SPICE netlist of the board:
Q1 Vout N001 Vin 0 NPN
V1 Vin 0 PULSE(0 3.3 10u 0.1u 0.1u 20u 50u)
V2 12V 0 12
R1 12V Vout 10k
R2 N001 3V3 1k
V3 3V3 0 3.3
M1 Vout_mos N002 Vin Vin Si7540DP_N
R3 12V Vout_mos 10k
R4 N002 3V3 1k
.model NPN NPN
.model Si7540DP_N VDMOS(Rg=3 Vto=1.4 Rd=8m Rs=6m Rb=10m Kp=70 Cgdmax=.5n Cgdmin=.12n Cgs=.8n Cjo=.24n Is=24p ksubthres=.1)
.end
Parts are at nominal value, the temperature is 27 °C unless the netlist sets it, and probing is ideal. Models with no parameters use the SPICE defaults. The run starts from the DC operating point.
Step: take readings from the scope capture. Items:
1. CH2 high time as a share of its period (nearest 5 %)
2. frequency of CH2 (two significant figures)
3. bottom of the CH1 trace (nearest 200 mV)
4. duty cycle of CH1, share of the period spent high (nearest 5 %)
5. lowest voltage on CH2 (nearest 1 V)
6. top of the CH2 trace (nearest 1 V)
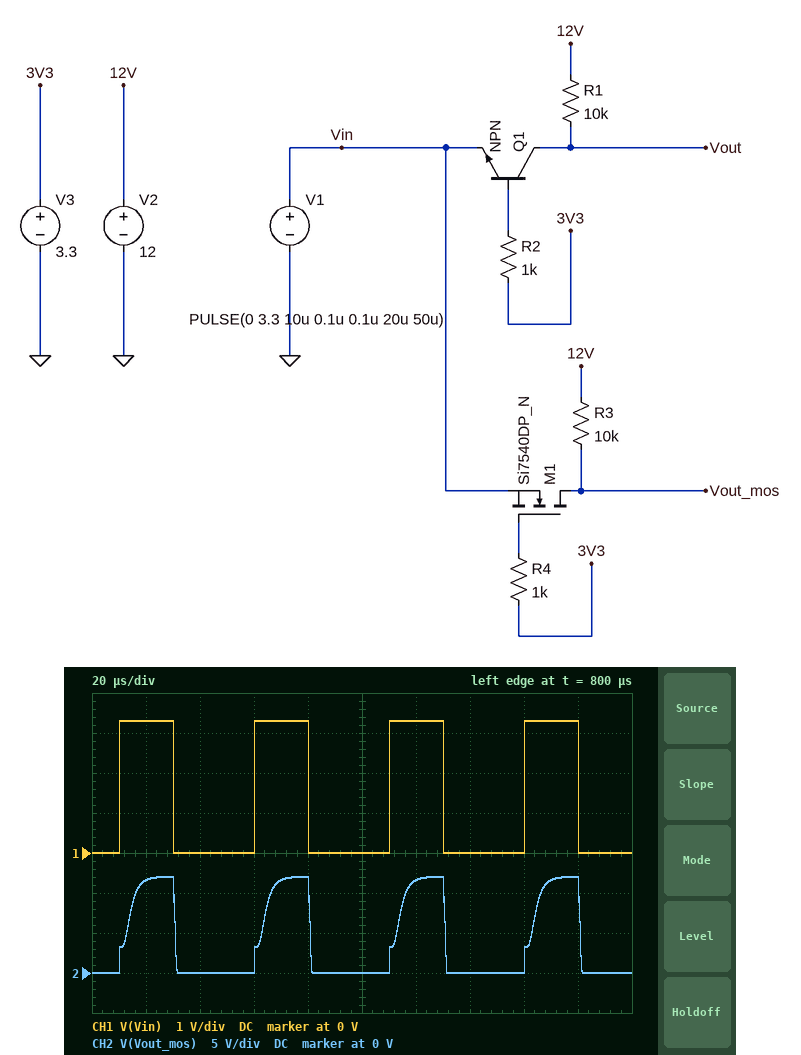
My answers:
35 %
20 kHz
0 V
40 %
0 V
12 V
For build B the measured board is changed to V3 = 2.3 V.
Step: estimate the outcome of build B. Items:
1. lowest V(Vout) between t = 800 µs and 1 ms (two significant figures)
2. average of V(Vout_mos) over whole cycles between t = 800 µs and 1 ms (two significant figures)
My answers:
27 mV
4.4 V
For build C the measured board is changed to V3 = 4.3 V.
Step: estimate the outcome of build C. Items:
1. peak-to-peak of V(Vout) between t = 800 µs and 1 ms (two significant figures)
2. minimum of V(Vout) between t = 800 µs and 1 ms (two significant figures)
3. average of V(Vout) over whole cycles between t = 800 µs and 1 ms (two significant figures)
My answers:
3.3 V
22 mV
1.4 V
